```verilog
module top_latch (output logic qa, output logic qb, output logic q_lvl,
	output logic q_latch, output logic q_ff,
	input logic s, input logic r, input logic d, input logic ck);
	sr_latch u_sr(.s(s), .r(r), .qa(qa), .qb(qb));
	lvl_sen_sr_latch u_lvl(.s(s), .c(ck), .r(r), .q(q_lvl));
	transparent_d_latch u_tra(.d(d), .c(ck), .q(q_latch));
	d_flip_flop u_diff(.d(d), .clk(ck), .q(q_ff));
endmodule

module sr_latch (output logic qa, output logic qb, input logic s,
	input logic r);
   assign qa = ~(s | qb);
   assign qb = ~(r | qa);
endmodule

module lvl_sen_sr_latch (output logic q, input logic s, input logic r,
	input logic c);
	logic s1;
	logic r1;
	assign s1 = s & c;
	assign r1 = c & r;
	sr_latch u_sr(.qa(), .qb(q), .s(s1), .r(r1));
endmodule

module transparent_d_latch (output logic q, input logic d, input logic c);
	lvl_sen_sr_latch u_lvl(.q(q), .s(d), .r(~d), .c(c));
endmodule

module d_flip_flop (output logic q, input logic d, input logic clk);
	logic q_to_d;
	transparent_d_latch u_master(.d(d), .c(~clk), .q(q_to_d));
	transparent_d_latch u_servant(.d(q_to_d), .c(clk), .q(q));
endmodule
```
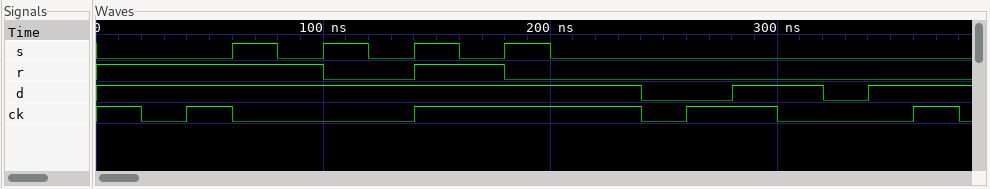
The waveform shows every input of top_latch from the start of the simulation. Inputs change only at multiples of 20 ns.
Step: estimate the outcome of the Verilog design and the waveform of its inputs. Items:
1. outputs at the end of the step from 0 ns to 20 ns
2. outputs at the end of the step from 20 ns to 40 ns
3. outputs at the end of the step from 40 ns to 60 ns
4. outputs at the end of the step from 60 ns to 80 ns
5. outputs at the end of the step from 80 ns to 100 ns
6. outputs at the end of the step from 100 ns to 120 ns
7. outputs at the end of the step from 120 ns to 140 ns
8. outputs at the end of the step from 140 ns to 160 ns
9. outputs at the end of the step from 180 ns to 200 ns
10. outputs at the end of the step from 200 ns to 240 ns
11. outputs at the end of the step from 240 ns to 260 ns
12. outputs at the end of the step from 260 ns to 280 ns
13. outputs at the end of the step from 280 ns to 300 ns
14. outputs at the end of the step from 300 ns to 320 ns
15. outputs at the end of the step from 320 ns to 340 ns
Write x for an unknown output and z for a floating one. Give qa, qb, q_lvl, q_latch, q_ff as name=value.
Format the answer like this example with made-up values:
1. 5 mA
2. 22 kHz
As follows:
1. qa=1, qb=0, q_lvl=0, q_latch=1, q_ff=x
2. qa=1, qb=0, q_lvl=0, q_latch=1, q_ff=x
3. qa=1, qb=0, q_lvl=0, q_latch=1, q_ff=1
4. qa=0, qb=0, q_lvl=0, q_latch=1, q_ff=1
5. qa=1, qb=0, q_lvl=0, q_latch=1, q_ff=1
6. qa=0, qb=1, q_lvl=0, q_latch=1, q_ff=1
7. qa=0, qb=1, q_lvl=0, q_latch=1, q_ff=1
8. qa=0, qb=0, q_lvl=0, q_latch=1, q_ff=1
9. qa=0, qb=1, q_lvl=1, q_latch=1, q_ff=1
10. qa=0, qb=1, q_lvl=1, q_latch=1, q_ff=1
11. qa=0, qb=1, q_lvl=1, q_latch=1, q_ff=1
12. qa=0, qb=1, q_lvl=1, q_latch=0, q_ff=0
13. qa=0, qb=1, q_lvl=1, q_latch=1, q_ff=0
14. qa=0, qb=1, q_lvl=1, q_latch=1, q_ff=0
15. qa=0, qb=1, q_lvl=1, q_latch=1, q_ff=0
